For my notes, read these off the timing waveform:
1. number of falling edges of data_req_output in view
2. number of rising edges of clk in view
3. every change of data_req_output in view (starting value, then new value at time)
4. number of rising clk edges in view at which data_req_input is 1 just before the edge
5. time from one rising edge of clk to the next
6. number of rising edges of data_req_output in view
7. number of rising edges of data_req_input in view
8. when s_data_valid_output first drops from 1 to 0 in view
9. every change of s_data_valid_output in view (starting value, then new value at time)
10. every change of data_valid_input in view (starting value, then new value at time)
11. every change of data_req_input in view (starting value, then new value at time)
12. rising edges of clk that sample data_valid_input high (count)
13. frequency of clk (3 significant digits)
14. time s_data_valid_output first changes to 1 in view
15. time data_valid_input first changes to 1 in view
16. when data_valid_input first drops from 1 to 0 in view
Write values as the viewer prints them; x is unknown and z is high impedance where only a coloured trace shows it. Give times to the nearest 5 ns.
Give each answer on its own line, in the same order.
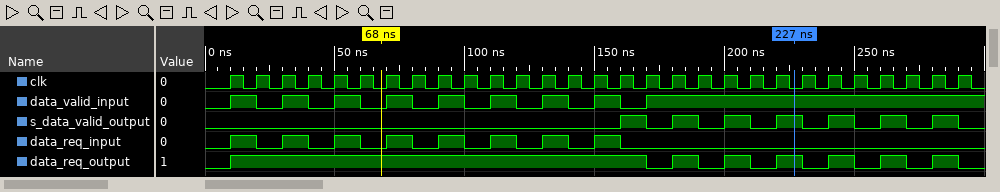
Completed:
7
29
0, 1 at 10 ns, 0 at 170 ns, 1 at 180 ns, 0 at 190 ns, 1 at 200 ns, 0 at 210 ns, 1 at 220 ns, 0 at 230 ns, 1 at 240 ns, 0 at 250 ns, 1 at 260 ns, 0 at 270 ns, 1 at 280 ns, 0 at 290 ns
8
10 ns
7
8
170 ns
0, 1 at 160 ns, 0 at 170 ns, 1 at 180 ns, 0 at 190 ns, 1 at 200 ns, 0 at 210 ns, 1 at 220 ns, 0 at 230 ns, 1 at 240 ns, 0 at 250 ns, 1 at 260 ns, 0 at 270 ns, 1 at 280 ns, 0 at 290 ns
0, 1 at 10 ns, 0 at 20 ns, 1 at 30 ns, 0 at 40 ns, 1 at 50 ns, 0 at 60 ns, 1 at 70 ns, 0 at 80 ns, 1 at 90 ns, 0 at 100 ns, 1 at 110 ns, 0 at 120 ns, 1 at 130 ns, 0 at 140 ns, 1 at 150 ns, 0 at 160 ns, 1 at 170 ns
0, 1 at 10 ns, 0 at 20 ns, 1 at 30 ns, 0 at 40 ns, 1 at 50 ns, 0 at 60 ns, 1 at 70 ns, 0 at 80 ns, 1 at 90 ns, 0 at 100 ns, 1 at 110 ns, 0 at 120 ns, 1 at 130 ns, 0 at 140 ns, 1 at 150 ns, 0 at 160 ns
20
100 MHz
160 ns
10 ns
20 ns
